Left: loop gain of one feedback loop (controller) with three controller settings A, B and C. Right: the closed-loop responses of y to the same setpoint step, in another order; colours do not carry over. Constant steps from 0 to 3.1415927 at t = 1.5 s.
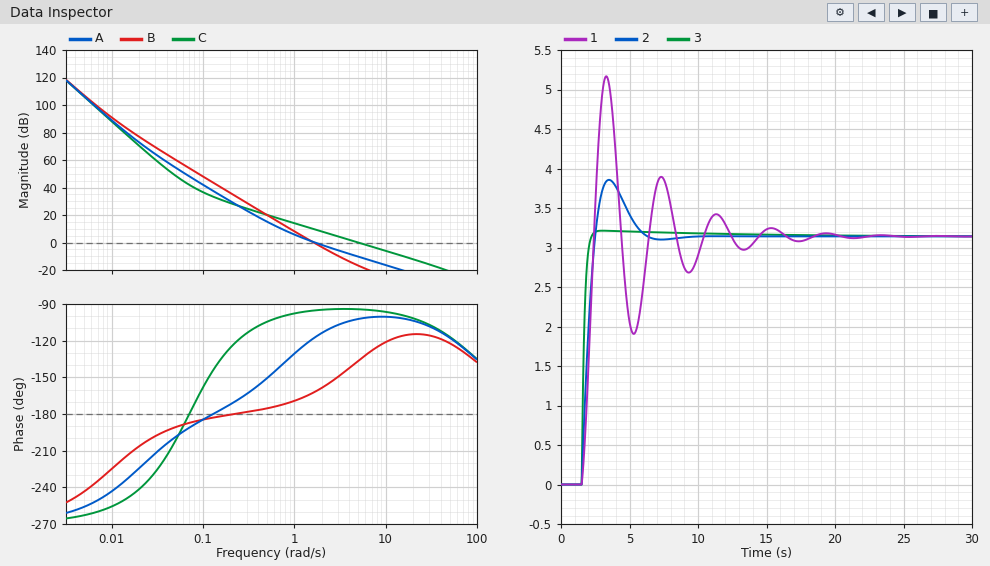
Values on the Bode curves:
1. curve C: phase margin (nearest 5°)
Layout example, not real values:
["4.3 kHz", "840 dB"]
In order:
["85°"]
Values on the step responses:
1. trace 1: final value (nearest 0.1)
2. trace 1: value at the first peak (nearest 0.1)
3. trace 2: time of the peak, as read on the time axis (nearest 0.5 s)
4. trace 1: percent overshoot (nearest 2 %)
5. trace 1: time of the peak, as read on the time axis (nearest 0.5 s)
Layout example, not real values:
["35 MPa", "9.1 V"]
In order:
["3.1", "5.2", "3.5 s", "64 %", "3.5 s"]
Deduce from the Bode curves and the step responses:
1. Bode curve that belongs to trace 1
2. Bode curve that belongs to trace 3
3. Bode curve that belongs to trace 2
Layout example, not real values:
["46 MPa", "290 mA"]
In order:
["B", "C", "A"]
